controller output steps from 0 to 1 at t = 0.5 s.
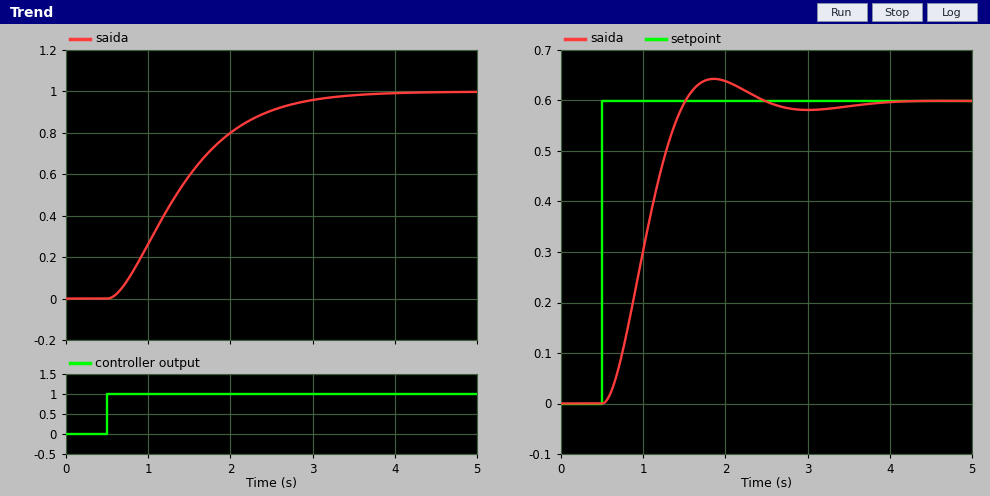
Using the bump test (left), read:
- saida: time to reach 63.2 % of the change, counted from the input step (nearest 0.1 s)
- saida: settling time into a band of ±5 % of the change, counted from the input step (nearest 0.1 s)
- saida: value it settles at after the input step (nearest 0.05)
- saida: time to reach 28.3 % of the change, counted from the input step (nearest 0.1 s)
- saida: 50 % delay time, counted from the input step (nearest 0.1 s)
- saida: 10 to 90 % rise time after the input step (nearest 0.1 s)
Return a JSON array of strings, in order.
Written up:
["1.1 s", "2.4 s", "1.00", "0.5 s", "0.8 s", "1.7 s"]
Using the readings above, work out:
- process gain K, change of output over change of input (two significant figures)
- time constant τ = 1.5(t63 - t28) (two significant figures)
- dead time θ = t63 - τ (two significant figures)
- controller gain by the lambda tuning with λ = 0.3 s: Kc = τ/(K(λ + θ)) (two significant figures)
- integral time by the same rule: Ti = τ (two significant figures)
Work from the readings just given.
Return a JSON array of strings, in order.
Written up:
["1.0", "0.90 s", "0.20 s", "1.8", "0.90 s"]
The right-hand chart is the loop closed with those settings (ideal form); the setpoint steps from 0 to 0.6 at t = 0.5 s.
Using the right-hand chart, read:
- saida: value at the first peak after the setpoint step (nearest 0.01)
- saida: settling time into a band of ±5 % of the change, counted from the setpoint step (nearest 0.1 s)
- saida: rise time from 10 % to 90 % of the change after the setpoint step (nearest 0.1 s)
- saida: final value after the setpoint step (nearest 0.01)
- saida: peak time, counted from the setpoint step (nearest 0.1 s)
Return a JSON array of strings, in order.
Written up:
["0.64", "1.6 s", "0.7 s", "0.60", "1.4 s"]
